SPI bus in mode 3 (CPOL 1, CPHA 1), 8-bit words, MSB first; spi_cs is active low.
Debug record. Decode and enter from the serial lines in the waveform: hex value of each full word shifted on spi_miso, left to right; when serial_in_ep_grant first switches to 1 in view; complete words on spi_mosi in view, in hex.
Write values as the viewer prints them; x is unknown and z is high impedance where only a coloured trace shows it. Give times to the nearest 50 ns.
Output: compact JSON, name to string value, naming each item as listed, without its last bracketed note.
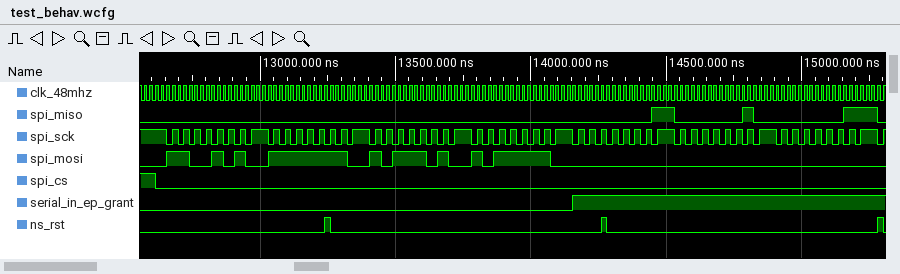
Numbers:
{"hex value of each full word shifted on spi_miso, left to right": "00, 00, 00, 00, 01, 02, 03", "when serial_in_ep_grant first switches to 1 in view": "14150 ns", "complete words on spi_mosi in view, in hex": "CA, FE, BA, BE, 00, 00, 00"}
